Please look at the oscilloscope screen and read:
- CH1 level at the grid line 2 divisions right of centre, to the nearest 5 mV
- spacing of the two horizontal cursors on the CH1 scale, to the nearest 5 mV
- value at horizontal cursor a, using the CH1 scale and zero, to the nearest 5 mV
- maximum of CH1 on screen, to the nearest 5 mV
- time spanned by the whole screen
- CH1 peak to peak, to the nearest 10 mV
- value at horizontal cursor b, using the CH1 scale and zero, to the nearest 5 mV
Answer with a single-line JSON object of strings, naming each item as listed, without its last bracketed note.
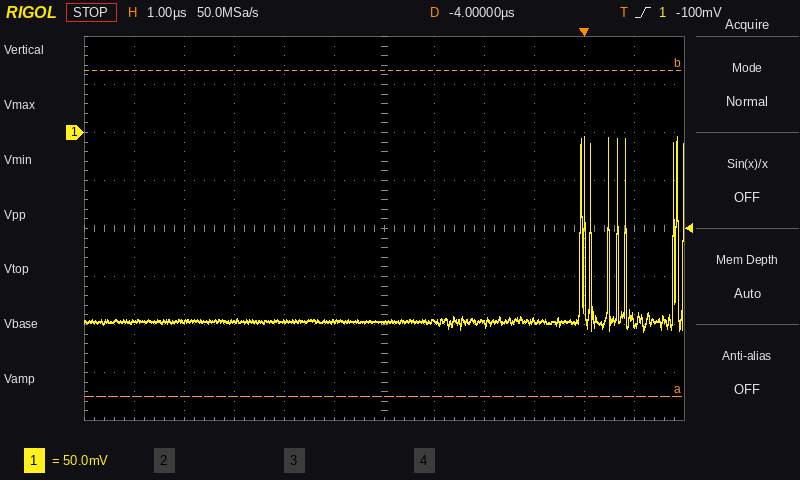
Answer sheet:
{"CH1 level at the grid line 2 divisions right of centre, to the nearest 5 mV": "-200 mV", "spacing of the two horizontal cursors on the CH1 scale, to the nearest 5 mV": "340 mV", "value at horizontal cursor a, using the CH1 scale and zero, to the nearest 5 mV": "-275 mV", "maximum of CH1 on screen, to the nearest 5 mV": "-5 mV", "time spanned by the whole screen": "12 µs", "CH1 peak to peak, to the nearest 10 mV": "200 mV", "value at horizontal cursor b, using the CH1 scale and zero, to the nearest 5 mV": "65 mV"}
